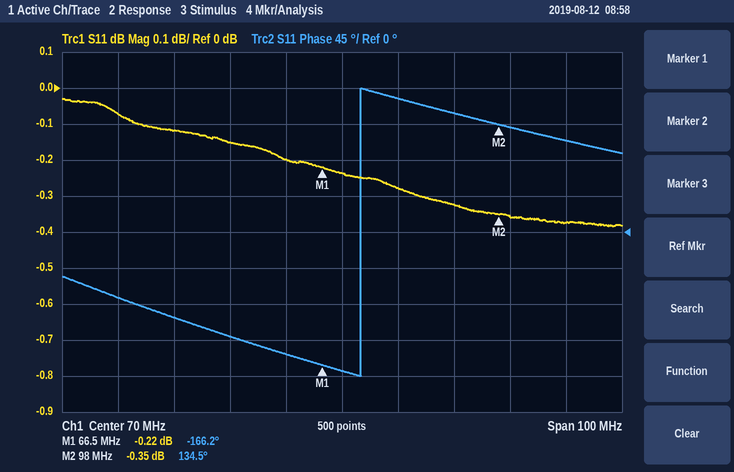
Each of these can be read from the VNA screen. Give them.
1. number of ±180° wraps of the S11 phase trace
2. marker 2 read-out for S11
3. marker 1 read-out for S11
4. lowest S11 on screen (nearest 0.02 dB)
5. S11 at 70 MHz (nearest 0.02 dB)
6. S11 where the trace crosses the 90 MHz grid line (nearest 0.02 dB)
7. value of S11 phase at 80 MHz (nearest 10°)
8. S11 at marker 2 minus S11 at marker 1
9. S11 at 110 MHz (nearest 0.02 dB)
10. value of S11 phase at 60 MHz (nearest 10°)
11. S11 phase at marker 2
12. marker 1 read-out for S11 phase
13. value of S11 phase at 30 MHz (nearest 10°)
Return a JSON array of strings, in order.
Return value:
["1", "-0.35 dB", "-0.22 dB", "-0.38 dB", "-0.24 dB", "-0.32 dB", "170°", "-0.13 dB", "-0.38 dB", "-150°", "134.5°", "-166.2°", "-80°"]
